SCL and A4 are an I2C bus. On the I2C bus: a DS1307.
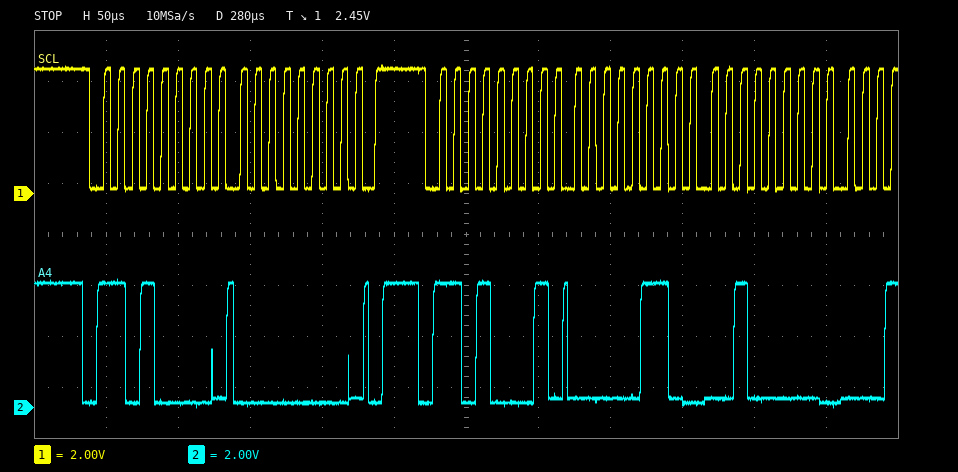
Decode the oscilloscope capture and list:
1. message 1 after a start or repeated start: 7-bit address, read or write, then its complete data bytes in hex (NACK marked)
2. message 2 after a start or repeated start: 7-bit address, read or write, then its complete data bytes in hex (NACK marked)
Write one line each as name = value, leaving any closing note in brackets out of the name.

message 1 after a start or repeated start: 7-bit address, read or write, then its complete data bytes in hex = 0x68 write: 00
message 2 after a start or repeated start: 7-bit address, read or write, then its complete data bytes in hex = 0x68 read: 06 20
